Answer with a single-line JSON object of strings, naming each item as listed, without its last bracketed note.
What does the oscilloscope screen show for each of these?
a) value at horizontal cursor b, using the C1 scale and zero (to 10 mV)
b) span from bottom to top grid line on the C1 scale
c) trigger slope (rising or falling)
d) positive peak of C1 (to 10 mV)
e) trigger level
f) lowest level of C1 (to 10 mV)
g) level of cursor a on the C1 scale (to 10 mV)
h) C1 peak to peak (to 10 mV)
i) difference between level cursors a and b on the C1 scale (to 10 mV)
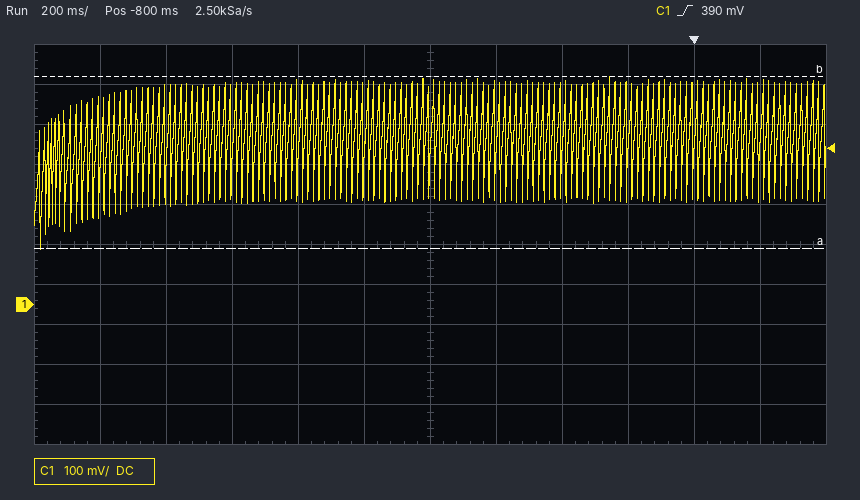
{"value at horizontal cursor b, using the C1 scale and zero": "570 mV", "span from bottom to top grid line on the C1 scale": "1 V", "trigger slope": "rising", "positive peak of C1": "570 mV", "trigger level": "390 mV", "lowest level of C1": "140 mV", "level of cursor a on the C1 scale": "140 mV", "C1 peak to peak": "430 mV", "difference between level cursors a and b on the C1 scale": "430 mV"}
